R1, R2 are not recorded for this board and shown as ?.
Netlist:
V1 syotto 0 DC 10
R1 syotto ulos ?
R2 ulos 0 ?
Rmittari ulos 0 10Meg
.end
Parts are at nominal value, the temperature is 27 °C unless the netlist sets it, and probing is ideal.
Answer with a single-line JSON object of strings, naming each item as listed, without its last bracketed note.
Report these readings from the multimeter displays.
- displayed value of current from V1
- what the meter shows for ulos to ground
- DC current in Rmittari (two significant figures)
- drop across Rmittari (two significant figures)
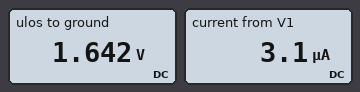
{"displayed value of current from V1": "3.1 µA", "what the meter shows for ulos to ground": "1.642 V", "DC current in Rmittari": "160 nA", "drop across Rmittari": "1.6 V"}
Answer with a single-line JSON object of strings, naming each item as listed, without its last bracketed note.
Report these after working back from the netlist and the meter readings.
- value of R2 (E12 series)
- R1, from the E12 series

{"value of R2": "560 kΩ", "R1, from the E12 series": "2.7 MΩ"}
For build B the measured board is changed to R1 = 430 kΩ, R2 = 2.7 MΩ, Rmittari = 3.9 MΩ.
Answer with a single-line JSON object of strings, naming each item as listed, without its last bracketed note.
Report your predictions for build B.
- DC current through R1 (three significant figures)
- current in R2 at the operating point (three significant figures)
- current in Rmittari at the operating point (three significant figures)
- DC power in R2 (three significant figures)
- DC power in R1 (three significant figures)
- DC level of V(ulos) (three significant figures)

{"DC current through R1": "4.94 µA", "current in R2 at the operating point": "2.92 µA", "current in Rmittari at the operating point": "2.02 µA", "DC power in R2": "23.0 µW", "DC power in R1": "10.5 µW", "DC level of V(ulos)": "7.88 V"}
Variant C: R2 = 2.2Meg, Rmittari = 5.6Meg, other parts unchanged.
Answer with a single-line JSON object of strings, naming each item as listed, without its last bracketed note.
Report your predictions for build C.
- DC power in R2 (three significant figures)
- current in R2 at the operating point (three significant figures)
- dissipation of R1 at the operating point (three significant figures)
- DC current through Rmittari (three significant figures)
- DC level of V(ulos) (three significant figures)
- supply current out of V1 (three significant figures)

{"DC power in R2": "6.19 µW", "current in R2 at the operating point": "1.68 µA", "dissipation of R1 at the operating point": "14.7 µW", "DC current through Rmittari": "659 nA", "DC level of V(ulos)": "3.69 V", "supply current out of V1": "2.34 µA"}
